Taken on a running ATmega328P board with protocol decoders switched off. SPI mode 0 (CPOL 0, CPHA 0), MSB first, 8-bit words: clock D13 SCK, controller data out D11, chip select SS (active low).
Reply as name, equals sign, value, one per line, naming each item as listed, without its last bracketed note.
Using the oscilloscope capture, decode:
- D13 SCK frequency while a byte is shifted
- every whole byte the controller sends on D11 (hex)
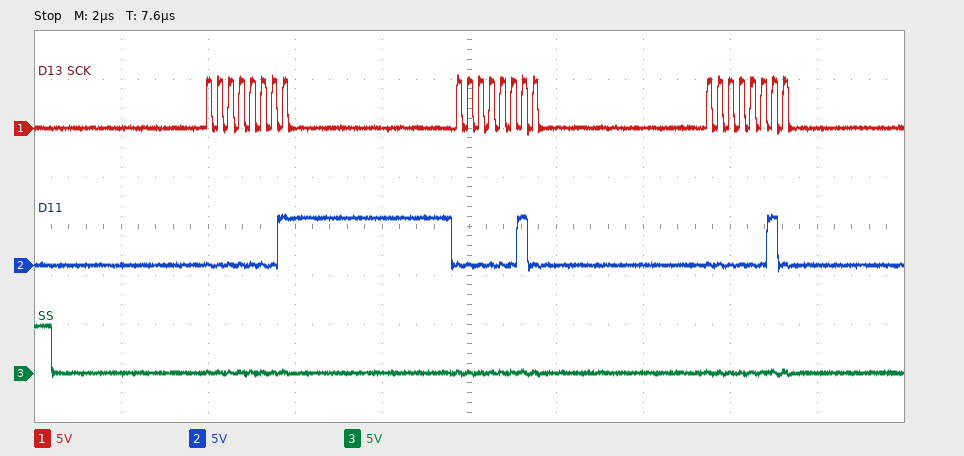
D13 SCK frequency while a byte is shifted = 4 MHz
every whole byte the controller sends on D11 = 01 02 02
